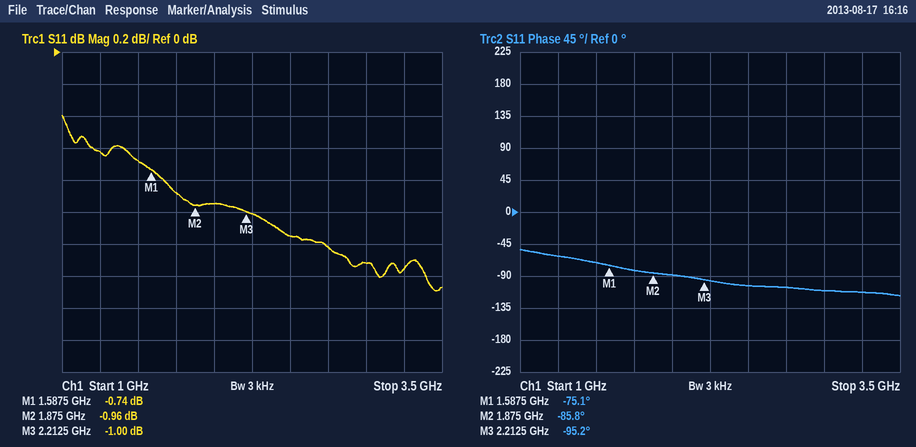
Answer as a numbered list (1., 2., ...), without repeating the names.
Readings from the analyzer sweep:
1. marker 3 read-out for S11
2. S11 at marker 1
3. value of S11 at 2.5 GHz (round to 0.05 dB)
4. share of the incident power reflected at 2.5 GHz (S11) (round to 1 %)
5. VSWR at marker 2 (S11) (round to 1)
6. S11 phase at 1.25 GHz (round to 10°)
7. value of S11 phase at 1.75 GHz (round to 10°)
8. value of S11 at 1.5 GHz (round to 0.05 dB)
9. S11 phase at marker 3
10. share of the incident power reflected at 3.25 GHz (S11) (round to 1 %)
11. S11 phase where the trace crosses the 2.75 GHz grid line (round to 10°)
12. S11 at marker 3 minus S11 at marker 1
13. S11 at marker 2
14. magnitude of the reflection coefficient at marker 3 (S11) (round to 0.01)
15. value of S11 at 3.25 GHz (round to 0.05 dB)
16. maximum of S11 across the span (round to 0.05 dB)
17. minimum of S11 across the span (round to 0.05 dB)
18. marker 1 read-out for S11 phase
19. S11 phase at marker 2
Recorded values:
1. -1.00 dB
2. -0.74 dB
3. -1.15 dB
4. 77 %
5. 18
6. -60°
7. -80°
8. -0.70 dB
9. -95.2°
10. 73 %
11. -110°
12. -0.26 dB
13. -0.96 dB
14. 0.89
15. -1.35 dB
16. -0.40 dB
17. -1.50 dB
18. -75.1°
19. -85.8°
